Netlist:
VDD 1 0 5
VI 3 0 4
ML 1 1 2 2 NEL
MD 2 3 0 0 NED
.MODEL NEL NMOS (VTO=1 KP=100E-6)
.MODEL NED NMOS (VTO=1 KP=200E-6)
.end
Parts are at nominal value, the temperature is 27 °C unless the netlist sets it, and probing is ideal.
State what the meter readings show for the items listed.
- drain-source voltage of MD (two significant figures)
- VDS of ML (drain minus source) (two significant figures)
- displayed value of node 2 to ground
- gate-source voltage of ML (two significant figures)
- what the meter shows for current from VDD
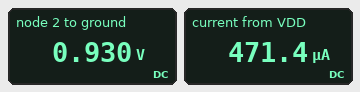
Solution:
930 mV
4.1 V
0.930 V
4.1 V
471.4 µA
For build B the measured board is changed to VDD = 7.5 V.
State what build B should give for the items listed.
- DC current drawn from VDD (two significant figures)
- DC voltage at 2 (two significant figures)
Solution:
860 µA
2.4 V
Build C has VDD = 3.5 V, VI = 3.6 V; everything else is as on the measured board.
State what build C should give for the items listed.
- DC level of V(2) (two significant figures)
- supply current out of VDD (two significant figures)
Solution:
440 mV
210 µA
